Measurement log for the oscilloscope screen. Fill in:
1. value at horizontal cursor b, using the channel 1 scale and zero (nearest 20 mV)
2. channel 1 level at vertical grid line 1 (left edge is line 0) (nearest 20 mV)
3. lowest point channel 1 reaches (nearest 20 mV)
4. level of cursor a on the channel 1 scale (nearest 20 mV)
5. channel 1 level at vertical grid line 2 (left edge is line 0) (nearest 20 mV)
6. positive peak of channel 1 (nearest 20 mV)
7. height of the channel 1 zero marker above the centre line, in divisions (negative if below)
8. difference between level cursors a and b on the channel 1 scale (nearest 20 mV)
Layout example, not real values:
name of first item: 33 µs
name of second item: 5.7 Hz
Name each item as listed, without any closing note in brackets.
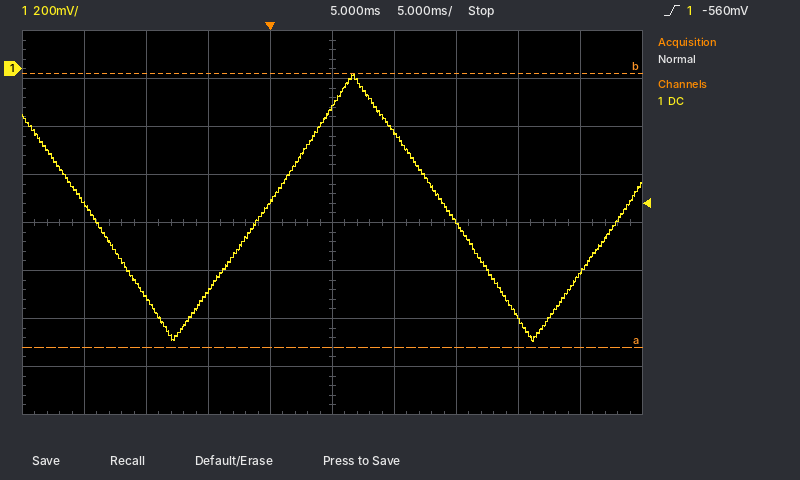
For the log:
value at horizontal cursor b, using the channel 1 scale and zero: -20 mV
channel 1 level at vertical grid line 1 (left edge is line 0): -560 mV
lowest point channel 1 reaches: -1.14 V
level of cursor a on the channel 1 scale: -1.16 V
channel 1 level at vertical grid line 2 (left edge is line 0): -940 mV
positive peak of channel 1: -20 mV
height of the channel 1 zero marker above the centre line, in divisions: +3.2 div
difference between level cursors a and b on the channel 1 scale: 1.14 V
